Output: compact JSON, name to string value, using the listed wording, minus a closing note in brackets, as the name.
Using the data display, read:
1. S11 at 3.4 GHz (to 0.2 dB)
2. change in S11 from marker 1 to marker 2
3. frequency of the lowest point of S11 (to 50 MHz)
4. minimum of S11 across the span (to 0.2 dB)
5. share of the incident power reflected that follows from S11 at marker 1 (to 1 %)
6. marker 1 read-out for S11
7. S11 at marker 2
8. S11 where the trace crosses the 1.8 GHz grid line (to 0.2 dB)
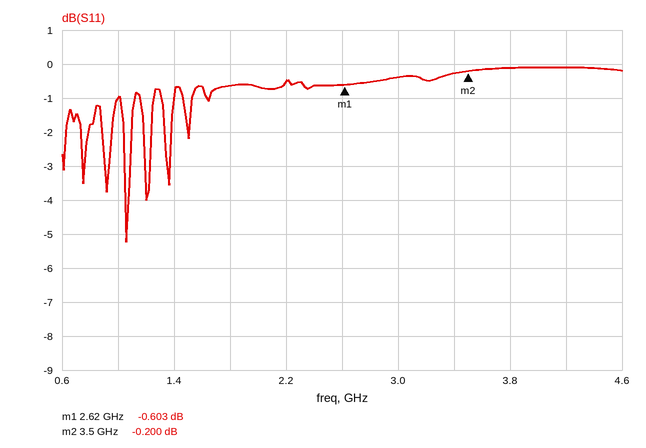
{"S11 at 3.4 GHz": "-0.2 dB", "change in S11 from marker 1 to marker 2": "0.403 dB", "frequency of the lowest point of S11": "1.05 GHz", "minimum of S11 across the span": "-5.2 dB", "share of the incident power reflected that follows from S11 at marker 1": "87 %", "marker 1 read-out for S11": "-0.603 dB", "S11 at marker 2": "-0.200 dB", "S11 where the trace crosses the 1.8 GHz grid line": "-0.6 dB"}
